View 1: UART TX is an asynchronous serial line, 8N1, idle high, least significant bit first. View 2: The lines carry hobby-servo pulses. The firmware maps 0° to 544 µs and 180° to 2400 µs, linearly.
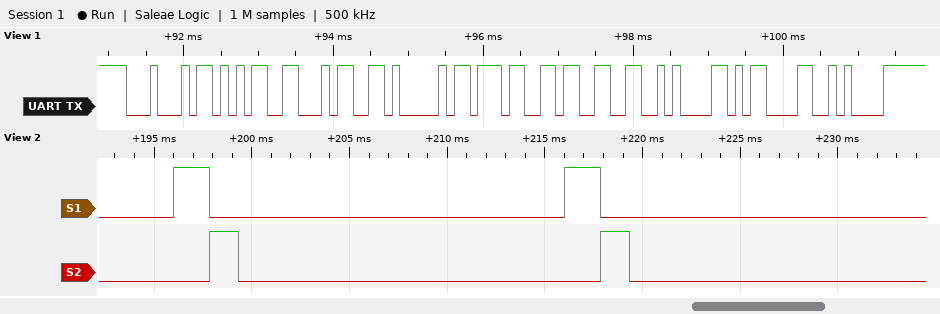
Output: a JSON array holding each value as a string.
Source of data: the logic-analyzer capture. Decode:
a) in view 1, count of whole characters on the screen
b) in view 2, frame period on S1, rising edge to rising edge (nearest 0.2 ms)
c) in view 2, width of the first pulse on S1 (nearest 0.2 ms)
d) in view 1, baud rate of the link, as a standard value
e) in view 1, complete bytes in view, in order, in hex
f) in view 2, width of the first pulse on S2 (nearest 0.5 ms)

["9", "20.0 ms", "1.8 ms", "9600 baud", "44 35 34 41 37 33 0A 0D 0A", "1.5 ms"]
